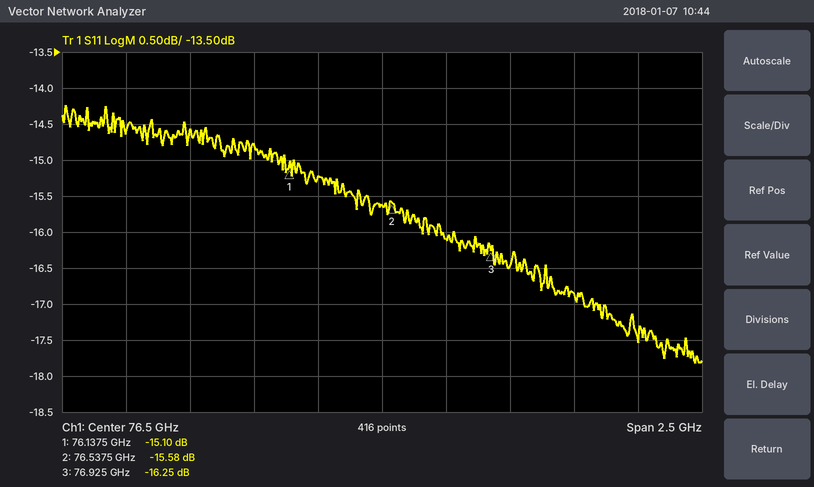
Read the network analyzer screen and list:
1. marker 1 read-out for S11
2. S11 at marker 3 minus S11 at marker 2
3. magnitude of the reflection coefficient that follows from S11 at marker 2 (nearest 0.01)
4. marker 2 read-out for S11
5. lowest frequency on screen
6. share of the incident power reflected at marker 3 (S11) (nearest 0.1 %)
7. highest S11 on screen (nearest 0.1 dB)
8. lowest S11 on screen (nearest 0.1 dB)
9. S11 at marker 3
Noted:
-15.10 dB
-0.67 dB
0.17
-15.58 dB
75.25 GHz
2.4 %
-14.2 dB
-17.8 dB
-16.25 dB
